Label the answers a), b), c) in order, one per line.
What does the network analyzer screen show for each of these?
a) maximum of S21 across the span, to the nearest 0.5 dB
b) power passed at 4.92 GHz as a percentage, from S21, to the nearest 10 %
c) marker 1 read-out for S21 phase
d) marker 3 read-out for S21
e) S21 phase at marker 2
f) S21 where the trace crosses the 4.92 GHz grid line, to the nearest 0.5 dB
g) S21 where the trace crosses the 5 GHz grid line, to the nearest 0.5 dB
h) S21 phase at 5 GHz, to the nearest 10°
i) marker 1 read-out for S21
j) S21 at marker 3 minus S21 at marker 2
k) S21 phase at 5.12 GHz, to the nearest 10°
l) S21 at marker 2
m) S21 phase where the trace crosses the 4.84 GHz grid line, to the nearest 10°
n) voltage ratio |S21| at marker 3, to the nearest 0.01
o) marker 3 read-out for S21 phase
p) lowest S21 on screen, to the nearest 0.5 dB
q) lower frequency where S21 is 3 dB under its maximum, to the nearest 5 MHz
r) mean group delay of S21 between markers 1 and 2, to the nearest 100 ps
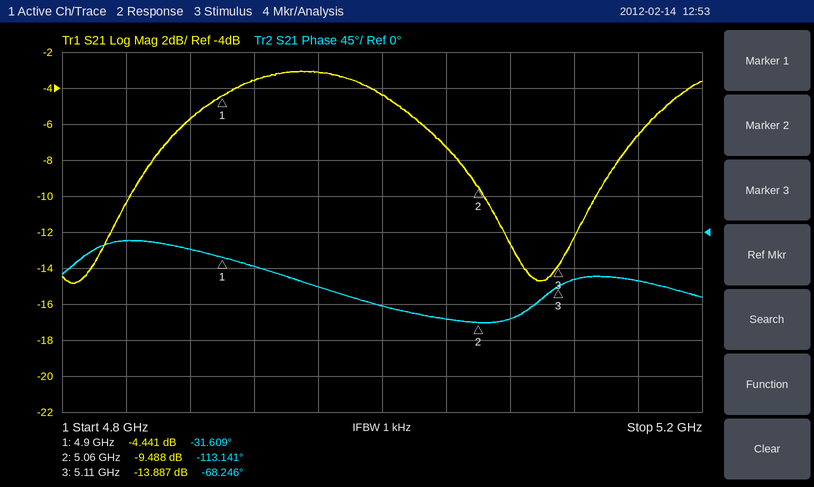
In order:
a) -3.0 dB
b) 40 %
c) -31.609°
d) -13.887 dB
e) -113.141°
f) -3.5 dB
g) -4.5 dB
h) -90°
i) -4.441 dB
j) -4.399 dB
k) -60°
l) -9.488 dB
m) -10°
n) 0.20
o) -68.246°
p) -15.0 dB
q) 4.875 GHz
r) 1.4 ns
